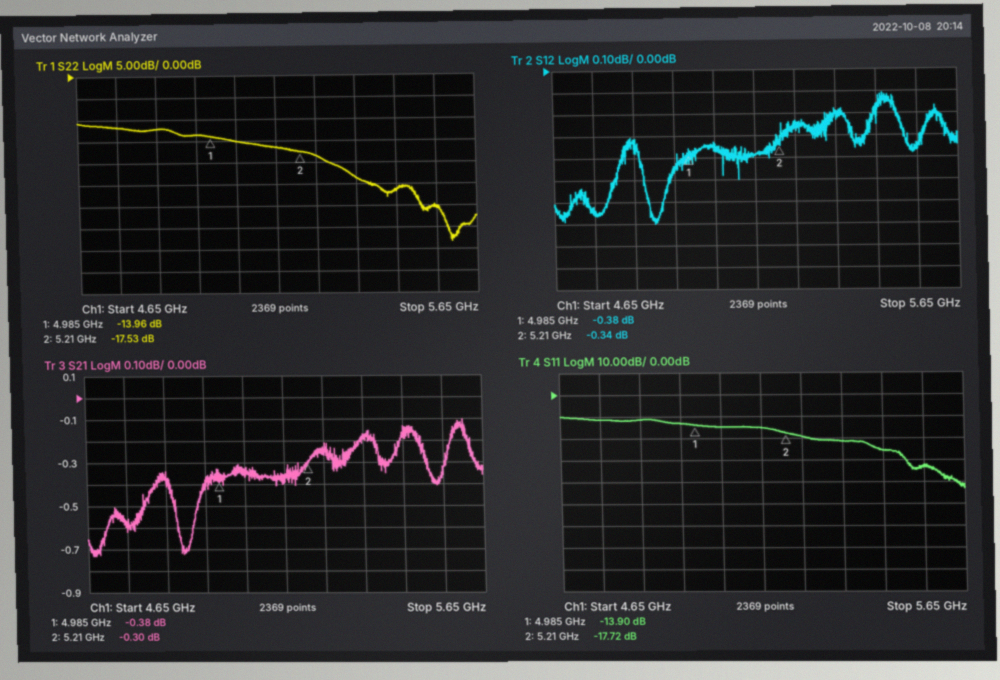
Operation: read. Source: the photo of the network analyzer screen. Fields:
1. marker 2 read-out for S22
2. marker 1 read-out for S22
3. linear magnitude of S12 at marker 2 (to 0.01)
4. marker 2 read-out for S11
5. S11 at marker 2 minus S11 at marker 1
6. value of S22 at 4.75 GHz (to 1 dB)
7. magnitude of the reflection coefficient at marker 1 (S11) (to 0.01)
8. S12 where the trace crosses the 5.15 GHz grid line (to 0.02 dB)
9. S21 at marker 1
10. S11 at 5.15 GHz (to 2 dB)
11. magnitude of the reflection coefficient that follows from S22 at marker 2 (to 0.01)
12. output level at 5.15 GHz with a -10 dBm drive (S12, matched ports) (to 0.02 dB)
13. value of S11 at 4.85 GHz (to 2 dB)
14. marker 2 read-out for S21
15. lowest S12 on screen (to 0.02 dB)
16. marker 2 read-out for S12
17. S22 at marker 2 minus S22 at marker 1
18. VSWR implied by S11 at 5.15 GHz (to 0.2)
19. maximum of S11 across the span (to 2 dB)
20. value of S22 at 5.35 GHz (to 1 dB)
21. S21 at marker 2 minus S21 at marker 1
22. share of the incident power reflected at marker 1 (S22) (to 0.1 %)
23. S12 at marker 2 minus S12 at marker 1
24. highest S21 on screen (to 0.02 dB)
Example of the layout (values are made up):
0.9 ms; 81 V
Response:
-17.53 dB; -13.96 dB; 0.96; -17.72 dB; -3.82 dB; -12 dB; 0.20; -0.38 dB; -0.38 dB; -16 dB; 0.13; -10.38 dBm; -12 dB; -0.30 dB; -0.70 dB; -0.34 dB; -3.57 dB; 1.4; -10 dB; -24 dB; 0.08 dB; 4.0 %; 0.04 dB; -0.10 dB
